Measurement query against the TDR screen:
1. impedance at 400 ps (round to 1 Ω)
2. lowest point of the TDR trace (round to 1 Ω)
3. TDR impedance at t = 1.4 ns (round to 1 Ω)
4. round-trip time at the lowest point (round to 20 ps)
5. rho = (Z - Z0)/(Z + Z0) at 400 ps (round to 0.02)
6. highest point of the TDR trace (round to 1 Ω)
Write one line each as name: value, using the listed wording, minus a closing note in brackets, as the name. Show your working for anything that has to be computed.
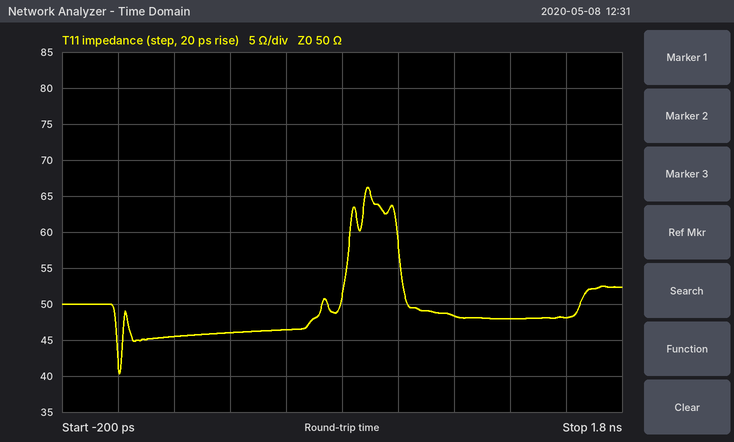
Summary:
impedance at 400 ps: 46 Ω
lowest point of the TDR trace: 40 Ω
TDR impedance at t = 1.4 ns: 48 Ω
round-trip time at the lowest point: 0 ps
rho = (Z - Z0)/(Z + Z0) at 400 ps: (46 − 50)/(46 + 50) ≈ -0.04
highest point of the TDR trace: 66 Ω
